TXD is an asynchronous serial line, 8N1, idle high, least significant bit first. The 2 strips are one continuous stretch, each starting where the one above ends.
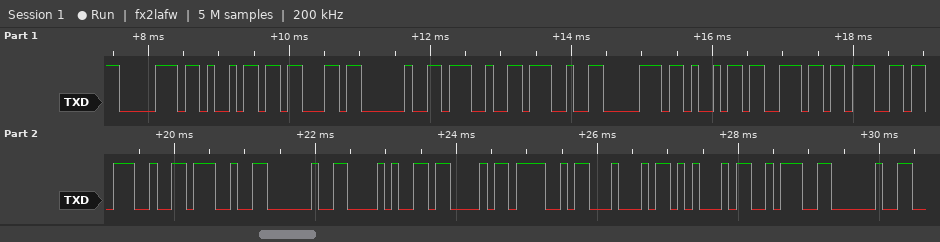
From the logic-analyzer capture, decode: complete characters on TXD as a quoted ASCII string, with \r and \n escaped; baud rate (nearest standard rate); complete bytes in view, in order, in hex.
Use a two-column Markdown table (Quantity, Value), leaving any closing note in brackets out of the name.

| Quantity | Value |
|---|---|
| complete characters on TXD as a quoted ASCII string, with \r and \n escaped | "pic ''ping'' (CODE: " |
| baud rate | 9600 baud |
| complete bytes in view, in order, in hex | 70 69 63 20 27 27 70 69 6E 67 27 27 20 28 43 4F 44 45 3A 20 |
